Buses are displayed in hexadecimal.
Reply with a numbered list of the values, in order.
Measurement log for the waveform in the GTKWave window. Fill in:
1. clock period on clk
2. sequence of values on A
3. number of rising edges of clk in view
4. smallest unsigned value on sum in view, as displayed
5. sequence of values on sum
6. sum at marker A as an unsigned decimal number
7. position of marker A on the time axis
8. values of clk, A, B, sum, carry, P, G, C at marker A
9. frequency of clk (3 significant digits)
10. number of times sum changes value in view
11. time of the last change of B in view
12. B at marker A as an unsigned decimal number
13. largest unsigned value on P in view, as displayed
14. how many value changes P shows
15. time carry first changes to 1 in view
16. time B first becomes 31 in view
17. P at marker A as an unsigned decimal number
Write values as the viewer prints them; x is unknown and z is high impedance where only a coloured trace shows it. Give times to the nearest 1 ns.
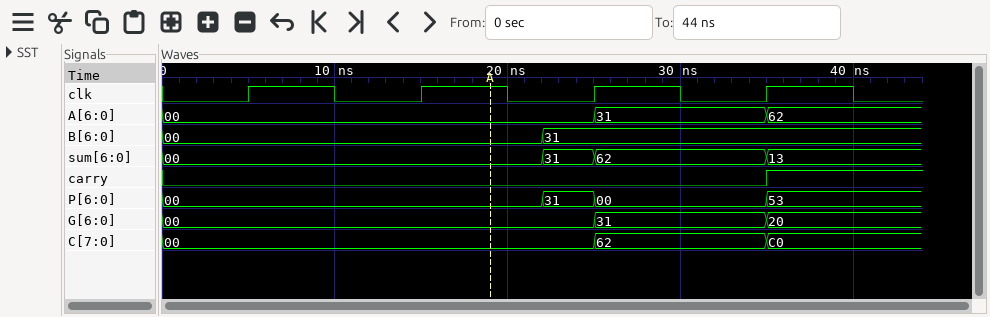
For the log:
1. 10 ns
2. 00, 31, 62
3. 4
4. 00
5. 00, 31, 62, 13
6. 0
7. 19 ns
8. clk=1, A=00, B=00, sum=00, carry=0, P=00, G=00, C=00
9. 100 MHz
10. 3
11. 22 ns
12. 0
13. 53
14. 3
15. 35 ns
16. 22 ns
17. 0
